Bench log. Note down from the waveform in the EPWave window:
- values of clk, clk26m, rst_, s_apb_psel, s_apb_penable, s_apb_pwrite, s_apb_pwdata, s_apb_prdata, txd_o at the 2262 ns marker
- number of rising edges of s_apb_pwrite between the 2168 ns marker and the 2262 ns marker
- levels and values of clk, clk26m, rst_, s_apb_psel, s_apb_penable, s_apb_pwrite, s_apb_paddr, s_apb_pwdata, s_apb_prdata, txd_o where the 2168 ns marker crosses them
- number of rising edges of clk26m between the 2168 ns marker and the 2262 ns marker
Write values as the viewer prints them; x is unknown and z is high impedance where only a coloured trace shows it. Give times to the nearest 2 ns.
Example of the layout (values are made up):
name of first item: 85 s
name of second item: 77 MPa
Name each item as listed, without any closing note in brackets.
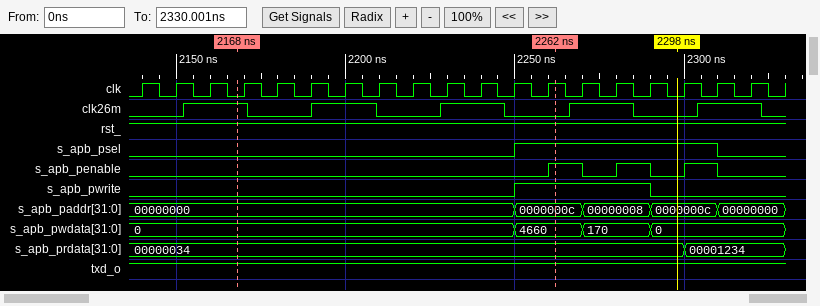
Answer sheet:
values of clk, clk26m, rst_, s_apb_psel, s_apb_penable, s_apb_pwrite, s_apb_pwdata, s_apb_prdata, txd_o at the 2262 ns marker: clk=1, clk26m=0, rst_=1, s_apb_psel=1, s_apb_penable=1, s_apb_pwrite=1, s_apb_pwdata=4660, s_apb_prdata=00000034, txd_o=1
number of rising edges of s_apb_pwrite between the 2168 ns marker and the 2262 ns marker: 1
levels and values of clk, clk26m, rst_, s_apb_psel, s_apb_penable, s_apb_pwrite, s_apb_paddr, s_apb_pwdata, s_apb_prdata, txd_o where the 2168 ns marker crosses them: clk=0, clk26m=1, rst_=1, s_apb_psel=0, s_apb_penable=0, s_apb_pwrite=0, s_apb_paddr=00000000, s_apb_pwdata=0, s_apb_prdata=00000034, txd_o=1
number of rising edges of clk26m between the 2168 ns marker and the 2262 ns marker: 2
